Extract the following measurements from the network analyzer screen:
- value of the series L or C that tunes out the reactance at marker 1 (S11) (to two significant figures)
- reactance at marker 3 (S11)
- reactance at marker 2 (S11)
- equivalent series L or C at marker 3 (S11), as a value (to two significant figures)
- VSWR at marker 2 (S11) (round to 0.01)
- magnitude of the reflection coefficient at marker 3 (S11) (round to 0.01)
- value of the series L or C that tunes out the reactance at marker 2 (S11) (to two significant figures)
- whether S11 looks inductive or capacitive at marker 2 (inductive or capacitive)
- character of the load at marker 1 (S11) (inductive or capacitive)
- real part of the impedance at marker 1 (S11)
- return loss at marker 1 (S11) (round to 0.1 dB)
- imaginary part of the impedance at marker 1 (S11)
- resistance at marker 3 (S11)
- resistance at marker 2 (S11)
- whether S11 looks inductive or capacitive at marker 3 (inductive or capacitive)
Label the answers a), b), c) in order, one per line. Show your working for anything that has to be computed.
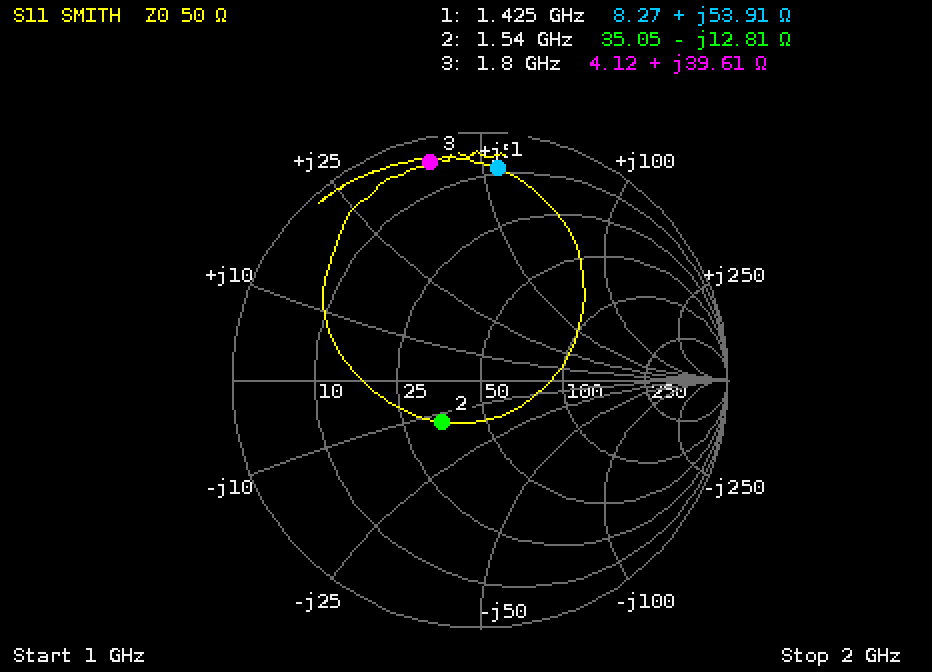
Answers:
a) C = 1/(2π × 1.425 GHz × 53.91 Ω) ≈ 2.1 pF
b) +39.61 Ω
c) -12.81 Ω
d) L = 39.61 Ω/(2π × 1.8 GHz) ≈ 3.5 nH
e) 1.59
f) 0.90
g) L = 12.81 Ω/(2π × 1.54 GHz) ≈ 1.3 nH
h) capacitive
i) inductive
j) 8.27 Ω
k) 1.3 dB
l) +53.91 Ω
m) 4.12 Ω
n) 35.05 Ω
o) inductive
